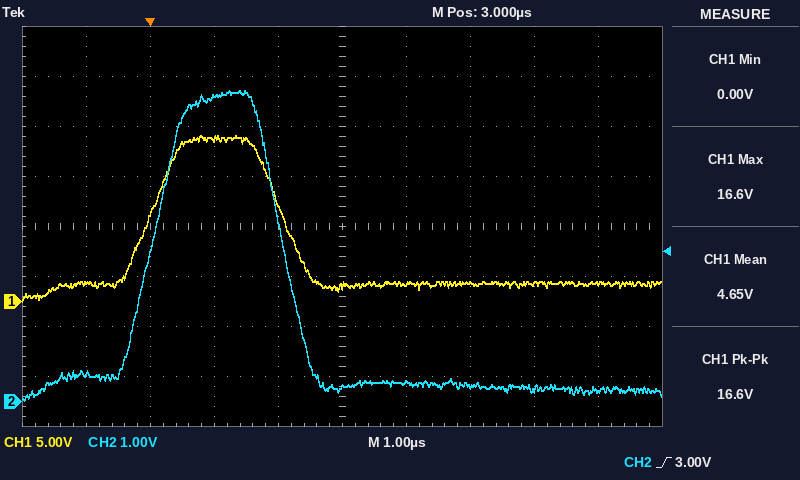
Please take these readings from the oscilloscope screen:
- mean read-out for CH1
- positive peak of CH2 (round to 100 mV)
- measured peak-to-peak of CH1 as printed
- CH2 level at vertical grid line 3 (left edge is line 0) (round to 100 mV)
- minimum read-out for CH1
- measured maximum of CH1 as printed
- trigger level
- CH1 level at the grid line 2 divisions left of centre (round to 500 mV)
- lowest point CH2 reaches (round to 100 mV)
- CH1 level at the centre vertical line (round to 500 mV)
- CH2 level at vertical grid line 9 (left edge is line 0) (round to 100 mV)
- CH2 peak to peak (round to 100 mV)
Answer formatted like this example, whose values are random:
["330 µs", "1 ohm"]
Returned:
["4.65 V", "6.2 V", "16.6 V", "6.1 V", "0.00 V", "16.6 V", "3.00 V", "16.5 V", "0.0 V", "1.5 V", "200 mV", "6.2 V"]
